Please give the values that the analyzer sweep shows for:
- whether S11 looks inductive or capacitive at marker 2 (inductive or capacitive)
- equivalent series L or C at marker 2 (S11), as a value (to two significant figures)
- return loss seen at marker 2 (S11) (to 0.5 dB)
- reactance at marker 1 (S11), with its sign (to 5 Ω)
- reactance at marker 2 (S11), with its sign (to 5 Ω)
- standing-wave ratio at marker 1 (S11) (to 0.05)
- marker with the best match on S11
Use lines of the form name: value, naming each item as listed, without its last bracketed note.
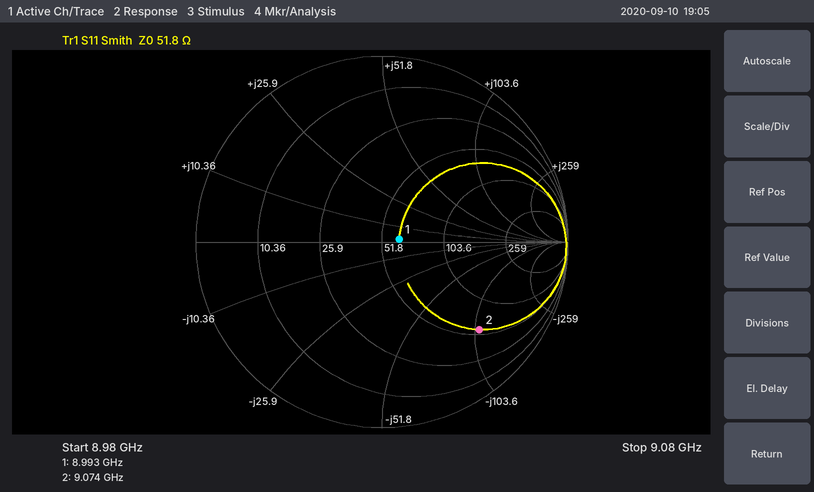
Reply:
whether S11 looks inductive or capacitive at marker 2: capacitive
equivalent series L or C at marker 2 (S11), as a value: 160 fF
return loss seen at marker 2 (S11): 3.0 dB
reactance at marker 1 (S11), with its sign: 0 Ω
reactance at marker 2 (S11), with its sign: -110 Ω
standing-wave ratio at marker 1 (S11): 1.20
marker with the best match on S11: marker 1
